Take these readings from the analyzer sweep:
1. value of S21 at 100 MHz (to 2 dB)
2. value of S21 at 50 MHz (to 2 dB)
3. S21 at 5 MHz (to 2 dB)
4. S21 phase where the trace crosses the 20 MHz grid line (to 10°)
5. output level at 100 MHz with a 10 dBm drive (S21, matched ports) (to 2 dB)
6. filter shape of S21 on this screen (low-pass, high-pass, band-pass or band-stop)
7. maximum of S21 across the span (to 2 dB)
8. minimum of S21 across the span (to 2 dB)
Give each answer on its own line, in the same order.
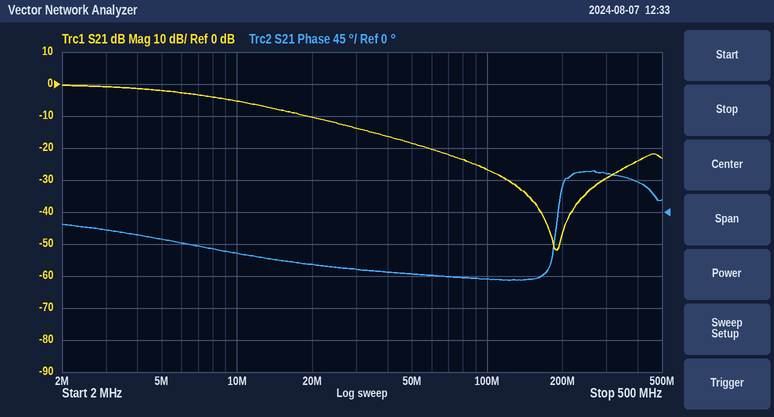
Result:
-26 dB
-18 dB
-2 dB
-70°
-16 dBm
low-pass
0 dB
-52 dB
